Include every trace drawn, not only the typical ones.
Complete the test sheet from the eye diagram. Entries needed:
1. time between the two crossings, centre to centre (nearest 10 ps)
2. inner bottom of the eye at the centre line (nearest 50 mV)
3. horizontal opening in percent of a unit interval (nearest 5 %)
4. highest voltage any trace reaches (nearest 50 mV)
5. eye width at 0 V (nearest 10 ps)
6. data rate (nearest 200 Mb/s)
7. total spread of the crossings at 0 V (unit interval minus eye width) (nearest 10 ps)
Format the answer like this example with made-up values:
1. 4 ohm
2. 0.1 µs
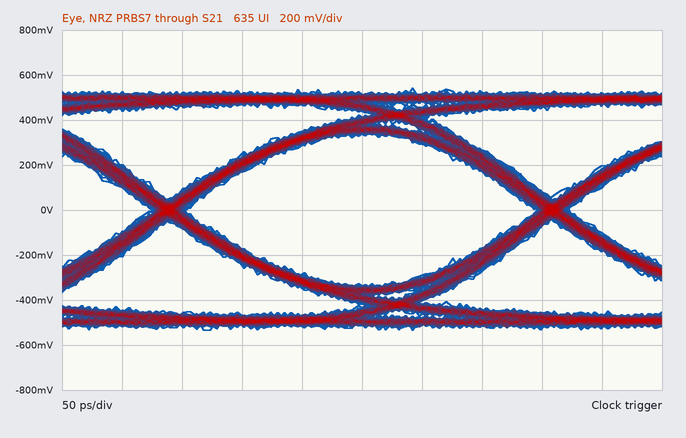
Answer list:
1. 320 ps
2. -350 mV
3. 90 %
4. 550 mV
5. 290 ps
6. 3.2 Gb/s
7. 30 ps
